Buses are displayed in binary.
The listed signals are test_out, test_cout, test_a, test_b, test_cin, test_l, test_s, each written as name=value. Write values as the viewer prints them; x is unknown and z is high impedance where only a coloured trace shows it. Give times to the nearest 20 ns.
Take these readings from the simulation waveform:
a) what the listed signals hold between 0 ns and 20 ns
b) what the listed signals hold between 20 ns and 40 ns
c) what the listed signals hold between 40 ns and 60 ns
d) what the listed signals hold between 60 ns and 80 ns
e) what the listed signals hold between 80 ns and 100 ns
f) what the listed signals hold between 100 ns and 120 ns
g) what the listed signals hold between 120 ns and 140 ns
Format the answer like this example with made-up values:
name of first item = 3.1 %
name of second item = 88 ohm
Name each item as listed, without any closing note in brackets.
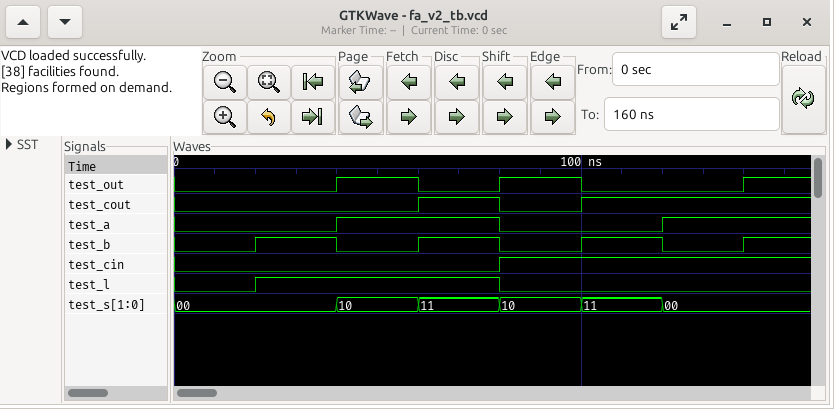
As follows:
what the listed signals hold between 0 ns and 20 ns = test_out=0, test_cout=0, test_a=0, test_b=0, test_cin=0, test_l=0, test_s=00
what the listed signals hold between 20 ns and 40 ns = test_out=0, test_cout=0, test_a=0, test_b=1, test_cin=0, test_l=1, test_s=00
what the listed signals hold between 40 ns and 60 ns = test_out=1, test_cout=0, test_a=1, test_b=0, test_cin=0, test_l=1, test_s=10
what the listed signals hold between 60 ns and 80 ns = test_out=0, test_cout=1, test_a=1, test_b=1, test_cin=0, test_l=1, test_s=11
what the listed signals hold between 80 ns and 100 ns = test_out=1, test_cout=0, test_a=0, test_b=0, test_cin=1, test_l=0, test_s=10
what the listed signals hold between 100 ns and 120 ns = test_out=0, test_cout=1, test_a=0, test_b=1, test_cin=1, test_l=0, test_s=11
what the listed signals hold between 120 ns and 140 ns = test_out=0, test_cout=1, test_a=1, test_b=0, test_cin=1, test_l=0, test_s=00
